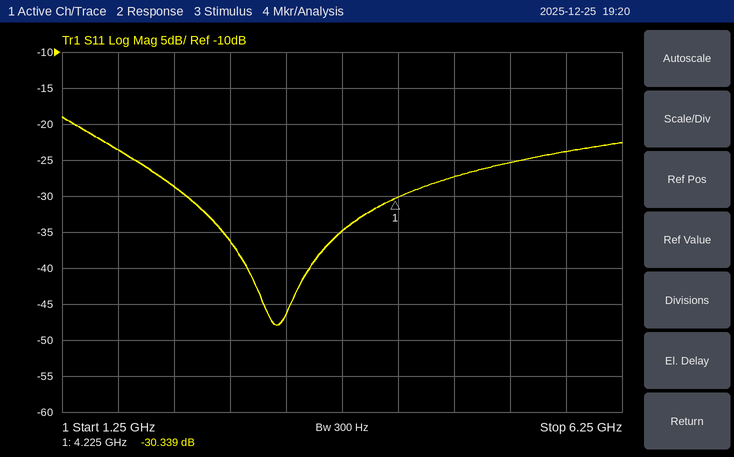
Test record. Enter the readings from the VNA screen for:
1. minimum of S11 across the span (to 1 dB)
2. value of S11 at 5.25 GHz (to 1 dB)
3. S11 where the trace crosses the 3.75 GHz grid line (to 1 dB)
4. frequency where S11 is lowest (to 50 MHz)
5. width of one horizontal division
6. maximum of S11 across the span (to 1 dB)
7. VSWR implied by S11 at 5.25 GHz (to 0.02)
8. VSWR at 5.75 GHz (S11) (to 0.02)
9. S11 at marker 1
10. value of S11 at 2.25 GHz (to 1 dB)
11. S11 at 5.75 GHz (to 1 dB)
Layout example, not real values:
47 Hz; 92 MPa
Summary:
-48 dB; -25 dB; -35 dB; 3.15 GHz; 500 MHz; -19 dB; 1.12; 1.14; -30.339 dB; -29 dB; -24 dB
